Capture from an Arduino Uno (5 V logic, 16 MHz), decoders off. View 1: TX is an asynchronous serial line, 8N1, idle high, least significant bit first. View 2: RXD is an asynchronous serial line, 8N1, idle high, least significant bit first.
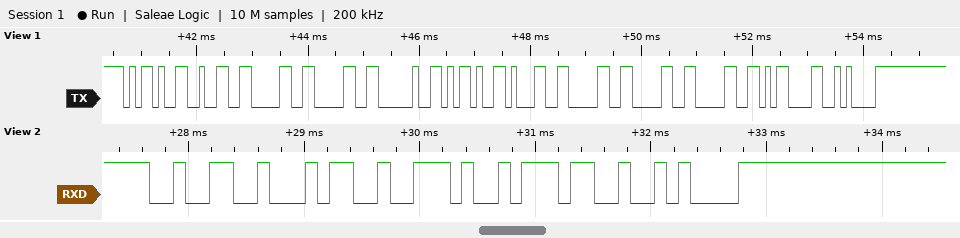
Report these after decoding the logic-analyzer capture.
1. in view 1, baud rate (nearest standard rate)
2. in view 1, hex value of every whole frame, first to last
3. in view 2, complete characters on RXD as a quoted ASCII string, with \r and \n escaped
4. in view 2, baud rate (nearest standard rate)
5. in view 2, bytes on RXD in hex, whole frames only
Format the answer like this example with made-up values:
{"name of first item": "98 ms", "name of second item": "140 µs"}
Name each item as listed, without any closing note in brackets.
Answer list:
{"in view 1, baud rate": "9600 baud", "in view 1, hex value of every whole frame, first to last": "2D 32 30 30 20 2D 31 30 30 30 0D 0A", "in view 2, complete characters on RXD as a quoted ASCII string, with \\r and \\n escaped": "\"24.7\\n\"", "in view 2, baud rate": "9600 baud", "in view 2, bytes on RXD in hex, whole frames only": "32 34 2E 37 0A"}
